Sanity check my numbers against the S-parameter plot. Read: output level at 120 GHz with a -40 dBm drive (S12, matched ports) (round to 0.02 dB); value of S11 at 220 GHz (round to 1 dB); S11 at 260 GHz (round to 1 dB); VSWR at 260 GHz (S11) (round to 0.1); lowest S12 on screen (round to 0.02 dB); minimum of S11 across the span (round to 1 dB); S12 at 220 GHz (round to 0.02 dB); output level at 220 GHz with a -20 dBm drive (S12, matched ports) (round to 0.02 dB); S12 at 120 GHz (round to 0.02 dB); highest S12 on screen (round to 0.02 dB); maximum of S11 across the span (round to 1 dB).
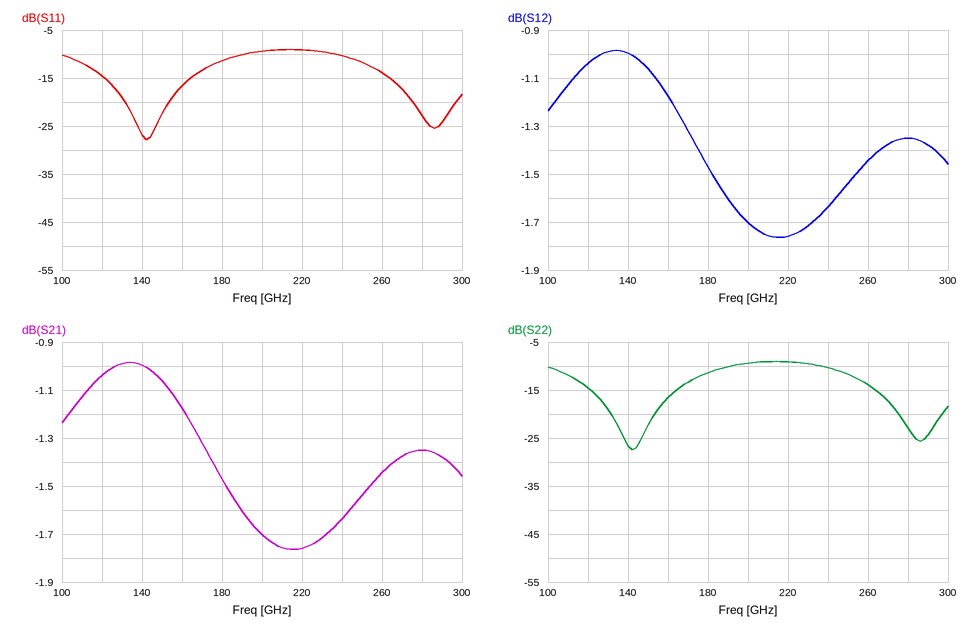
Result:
-41.04 dBm
-9 dB
-14 dB
1.5
-1.76 dB
-28 dB
-1.76 dB
-21.76 dBm
-1.04 dB
-0.98 dB
-9 dB
